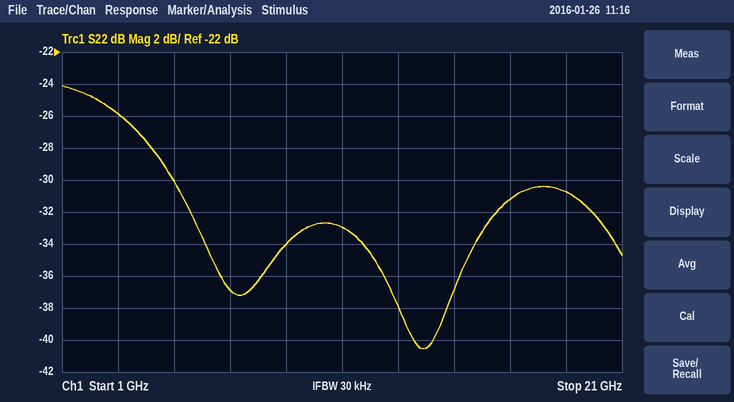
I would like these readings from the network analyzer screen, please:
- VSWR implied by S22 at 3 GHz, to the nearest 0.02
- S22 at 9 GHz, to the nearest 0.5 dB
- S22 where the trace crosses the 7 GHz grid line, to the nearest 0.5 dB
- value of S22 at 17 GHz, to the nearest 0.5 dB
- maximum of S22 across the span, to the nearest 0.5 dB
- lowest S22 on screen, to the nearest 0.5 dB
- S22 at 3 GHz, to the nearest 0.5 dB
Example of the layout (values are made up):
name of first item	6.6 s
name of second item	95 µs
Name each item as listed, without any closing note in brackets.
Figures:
VSWR implied by S22 at 3 GHz, to the nearest 0.02	1.10
S22 at 9 GHz, to the nearest 0.5 dB	-34.0 dB
S22 where the trace crosses the 7 GHz grid line, to the nearest 0.5 dB	-37.0 dB
value of S22 at 17 GHz, to the nearest 0.5 dB	-31.0 dB
maximum of S22 across the span, to the nearest 0.5 dB	-24.0 dB
lowest S22 on screen, to the nearest 0.5 dB	-40.5 dB
S22 at 3 GHz, to the nearest 0.5 dB	-26.0 dB
